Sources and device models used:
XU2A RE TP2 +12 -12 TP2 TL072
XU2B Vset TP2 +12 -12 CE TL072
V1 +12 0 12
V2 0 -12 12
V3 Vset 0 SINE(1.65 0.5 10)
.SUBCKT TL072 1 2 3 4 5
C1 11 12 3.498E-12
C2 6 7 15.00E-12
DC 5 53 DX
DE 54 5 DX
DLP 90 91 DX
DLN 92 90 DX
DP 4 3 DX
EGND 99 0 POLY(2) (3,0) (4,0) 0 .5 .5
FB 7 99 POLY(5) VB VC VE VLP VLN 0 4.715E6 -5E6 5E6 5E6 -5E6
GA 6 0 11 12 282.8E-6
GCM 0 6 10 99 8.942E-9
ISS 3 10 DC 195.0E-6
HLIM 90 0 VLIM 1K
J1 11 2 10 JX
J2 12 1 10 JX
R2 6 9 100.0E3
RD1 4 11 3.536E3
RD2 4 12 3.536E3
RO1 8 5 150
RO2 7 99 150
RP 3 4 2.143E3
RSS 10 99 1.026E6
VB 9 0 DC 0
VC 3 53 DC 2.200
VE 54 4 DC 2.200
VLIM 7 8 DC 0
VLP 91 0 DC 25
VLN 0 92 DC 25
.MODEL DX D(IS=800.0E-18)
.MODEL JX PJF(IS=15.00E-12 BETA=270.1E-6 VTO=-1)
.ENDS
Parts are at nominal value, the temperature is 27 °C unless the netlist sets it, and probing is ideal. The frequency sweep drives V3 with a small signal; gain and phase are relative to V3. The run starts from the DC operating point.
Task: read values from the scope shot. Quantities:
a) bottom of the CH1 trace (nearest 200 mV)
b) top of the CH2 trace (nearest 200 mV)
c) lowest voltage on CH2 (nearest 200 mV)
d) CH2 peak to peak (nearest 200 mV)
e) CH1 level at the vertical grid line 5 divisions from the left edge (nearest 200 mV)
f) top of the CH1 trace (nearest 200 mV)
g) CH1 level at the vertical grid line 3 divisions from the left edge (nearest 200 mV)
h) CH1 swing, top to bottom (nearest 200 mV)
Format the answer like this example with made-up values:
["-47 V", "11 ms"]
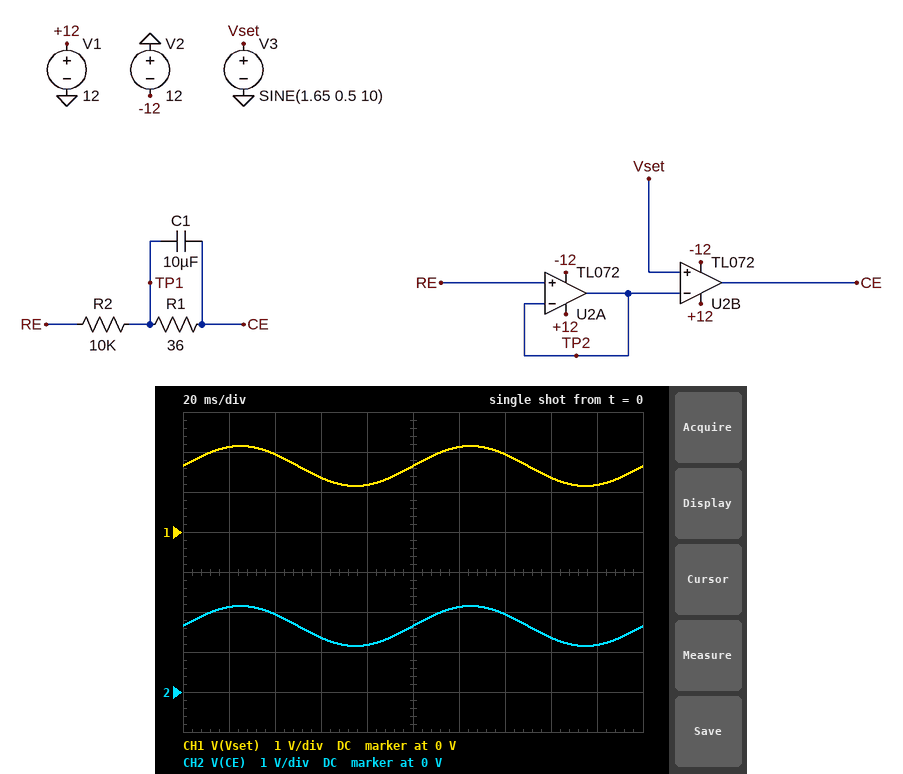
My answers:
["1.2 V", "2.2 V", "1.2 V", "1.0 V", "1.6 V", "2.2 V", "1.4 V", "1.0 V"]
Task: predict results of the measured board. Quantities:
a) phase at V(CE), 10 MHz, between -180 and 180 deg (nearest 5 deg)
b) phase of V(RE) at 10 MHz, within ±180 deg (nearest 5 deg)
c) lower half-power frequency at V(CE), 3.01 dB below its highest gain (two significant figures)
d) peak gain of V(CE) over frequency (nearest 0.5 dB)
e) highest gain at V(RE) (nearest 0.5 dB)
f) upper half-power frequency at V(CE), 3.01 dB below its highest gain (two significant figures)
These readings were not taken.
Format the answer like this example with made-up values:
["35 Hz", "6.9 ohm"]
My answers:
["-150 deg", "-150 deg", "3.0 MHz", "18.5 dB", "18.5 dB", "3.3 MHz"]
